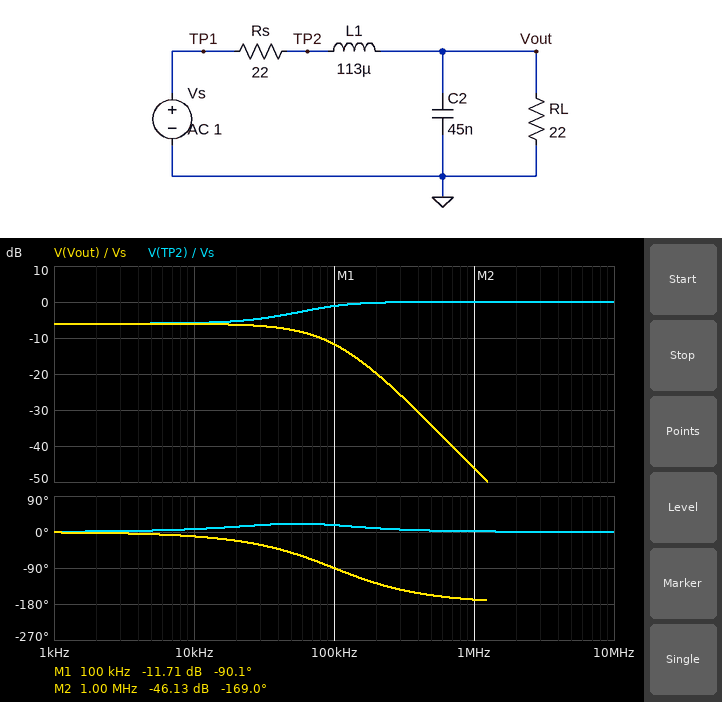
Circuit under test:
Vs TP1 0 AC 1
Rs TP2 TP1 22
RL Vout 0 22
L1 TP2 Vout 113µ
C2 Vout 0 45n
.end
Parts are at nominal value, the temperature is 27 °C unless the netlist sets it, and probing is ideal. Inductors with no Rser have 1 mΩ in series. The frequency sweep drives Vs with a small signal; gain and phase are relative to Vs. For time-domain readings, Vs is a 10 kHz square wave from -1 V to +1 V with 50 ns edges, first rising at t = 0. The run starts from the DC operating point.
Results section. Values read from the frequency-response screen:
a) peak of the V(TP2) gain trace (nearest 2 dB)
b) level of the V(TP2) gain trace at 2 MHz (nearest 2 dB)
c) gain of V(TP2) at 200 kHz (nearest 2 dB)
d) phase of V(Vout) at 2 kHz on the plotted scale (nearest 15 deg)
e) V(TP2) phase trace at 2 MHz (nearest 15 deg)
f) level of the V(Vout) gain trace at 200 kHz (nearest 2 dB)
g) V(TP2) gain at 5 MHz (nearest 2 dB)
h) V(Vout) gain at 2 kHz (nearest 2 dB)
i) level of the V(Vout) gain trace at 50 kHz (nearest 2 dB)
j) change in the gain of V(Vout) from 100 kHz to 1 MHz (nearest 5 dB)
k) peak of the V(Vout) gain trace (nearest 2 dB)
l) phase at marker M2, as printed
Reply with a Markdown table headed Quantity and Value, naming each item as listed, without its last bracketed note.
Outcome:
| Quantity | Value |
|---|---|
| peak of the V(TP2) gain trace | 0 dB |
| level of the V(TP2) gain trace at 2 MHz | 0 dB |
| gain of V(TP2) at 200 kHz | 0 dB |
| phase of V(Vout) at 2 kHz on the plotted scale | 0 deg |
| V(TP2) phase trace at 2 MHz | 0 deg |
| level of the V(Vout) gain trace at 200 kHz | -20 dB |
| V(TP2) gain at 5 MHz | 0 dB |
| V(Vout) gain at 2 kHz | -6 dB |
| level of the V(Vout) gain trace at 50 kHz | -8 dB |
| change in the gain of V(Vout) from 100 kHz to 1 MHz | -35 dB |
| peak of the V(Vout) gain trace | -6 dB |
| phase at marker M2, as printed | -169.0 deg |
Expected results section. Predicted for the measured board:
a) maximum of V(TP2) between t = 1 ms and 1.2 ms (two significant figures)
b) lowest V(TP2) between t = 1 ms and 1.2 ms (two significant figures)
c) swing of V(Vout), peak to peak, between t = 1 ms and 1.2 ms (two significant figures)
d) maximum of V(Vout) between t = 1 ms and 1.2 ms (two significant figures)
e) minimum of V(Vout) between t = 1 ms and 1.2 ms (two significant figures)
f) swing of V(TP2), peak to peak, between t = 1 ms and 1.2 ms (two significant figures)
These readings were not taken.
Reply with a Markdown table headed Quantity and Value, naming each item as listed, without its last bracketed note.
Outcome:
| Quantity | Value |
|---|---|
| maximum of V(TP2) between t = 1 ms and 1.2 ms | 1.5 V |
| lowest V(TP2) between t = 1 ms and 1.2 ms | -1.5 V |
| swing of V(Vout), peak to peak, between t = 1 ms and 1.2 ms | 1.0 V |
| maximum of V(Vout) between t = 1 ms and 1.2 ms | 500 mV |
| minimum of V(Vout) between t = 1 ms and 1.2 ms | -500 mV |
| swing of V(TP2), peak to peak, between t = 1 ms and 1.2 ms | 3.0 V |
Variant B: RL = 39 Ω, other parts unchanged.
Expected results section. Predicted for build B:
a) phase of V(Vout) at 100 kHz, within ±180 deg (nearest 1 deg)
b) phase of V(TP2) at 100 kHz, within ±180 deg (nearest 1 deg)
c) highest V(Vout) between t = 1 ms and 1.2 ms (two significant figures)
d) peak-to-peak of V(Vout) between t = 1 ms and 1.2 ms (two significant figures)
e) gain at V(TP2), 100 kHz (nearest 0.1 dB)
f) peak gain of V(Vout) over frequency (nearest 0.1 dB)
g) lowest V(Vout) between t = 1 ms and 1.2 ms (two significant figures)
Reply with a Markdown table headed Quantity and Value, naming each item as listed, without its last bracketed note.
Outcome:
| Quantity | Value |
|---|---|
| phase of V(Vout) at 100 kHz, within ±180 deg | -100 deg |
| phase of V(TP2) at 100 kHz, within ±180 deg | 19 deg |
| highest V(Vout) between t = 1 ms and 1.2 ms | 700 mV |
| peak-to-peak of V(Vout) between t = 1 ms and 1.2 ms | 1.4 V |
| gain at V(TP2), 100 kHz | -1.5 dB |
| peak gain of V(Vout) over frequency | -3.9 dB |
| lowest V(Vout) between t = 1 ms and 1.2 ms | -700 mV |
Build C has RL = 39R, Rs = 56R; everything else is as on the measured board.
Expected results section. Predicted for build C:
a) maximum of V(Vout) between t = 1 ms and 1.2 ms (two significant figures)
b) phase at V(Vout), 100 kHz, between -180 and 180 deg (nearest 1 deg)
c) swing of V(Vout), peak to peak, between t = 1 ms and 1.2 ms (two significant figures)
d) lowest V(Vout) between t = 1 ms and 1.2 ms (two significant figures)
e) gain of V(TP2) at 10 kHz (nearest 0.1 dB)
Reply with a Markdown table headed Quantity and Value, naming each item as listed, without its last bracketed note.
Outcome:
| Quantity | Value |
|---|---|
| maximum of V(Vout) between t = 1 ms and 1.2 ms | 430 mV |
| phase at V(Vout), 100 kHz, between -180 and 180 deg | -83 deg |
| swing of V(Vout), peak to peak, between t = 1 ms and 1.2 ms | 860 mV |
| lowest V(Vout) between t = 1 ms and 1.2 ms | -430 mV |
| gain of V(TP2) at 10 kHz | -7.8 dB |
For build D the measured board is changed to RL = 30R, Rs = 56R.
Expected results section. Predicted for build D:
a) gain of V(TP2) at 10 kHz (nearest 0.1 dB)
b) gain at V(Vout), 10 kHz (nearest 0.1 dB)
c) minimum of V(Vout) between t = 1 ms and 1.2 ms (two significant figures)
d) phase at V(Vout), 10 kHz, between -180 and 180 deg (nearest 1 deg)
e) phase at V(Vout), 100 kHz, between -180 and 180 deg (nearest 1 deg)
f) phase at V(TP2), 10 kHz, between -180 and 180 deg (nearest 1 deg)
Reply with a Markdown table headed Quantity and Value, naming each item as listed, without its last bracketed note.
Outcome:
| Quantity | Value |
|---|---|
| gain of V(TP2) at 10 kHz | -9.1 dB |
| gain at V(Vout), 10 kHz | -9.2 dB |
| minimum of V(Vout) between t = 1 ms and 1.2 ms | -360 mV |
| phase at V(Vout), 10 kHz, between -180 and 180 deg | -8 deg |
| phase at V(Vout), 100 kHz, between -180 and 180 deg | -78 deg |
| phase at V(TP2), 10 kHz, between -180 and 180 deg | 6 deg |
